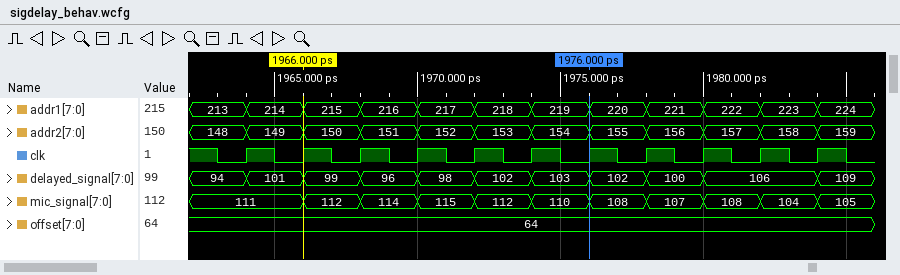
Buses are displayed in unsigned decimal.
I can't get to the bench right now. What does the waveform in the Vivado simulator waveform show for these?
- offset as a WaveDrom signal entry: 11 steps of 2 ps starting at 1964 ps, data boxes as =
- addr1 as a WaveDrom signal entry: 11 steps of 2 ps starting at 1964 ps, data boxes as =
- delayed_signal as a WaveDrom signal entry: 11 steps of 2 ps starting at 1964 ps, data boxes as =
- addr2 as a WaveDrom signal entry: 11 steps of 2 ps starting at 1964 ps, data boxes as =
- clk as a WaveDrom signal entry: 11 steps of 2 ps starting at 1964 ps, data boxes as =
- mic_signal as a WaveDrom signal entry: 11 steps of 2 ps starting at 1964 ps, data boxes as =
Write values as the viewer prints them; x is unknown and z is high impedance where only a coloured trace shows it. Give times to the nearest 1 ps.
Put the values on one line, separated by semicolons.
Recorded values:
{name: 'offset', wave: '=..........', data: '64'}; {name: 'addr1', wave: '===========', data: '214 215 216 217 218 219 220 221 222 223 224'}; {name: 'delayed_signal', wave: '=========.=', data: '101 99 96 98 102 103 102 100 106 109'}; {name: 'addr2', wave: '===========', data: '149 150 151 152 153 154 155 156 157 158 159'}; {name: 'clk', wave: 'p..........'}; {name: 'mic_signal', wave: '===========', data: '111 112 114 115 112 110 108 107 108 104 105'}
